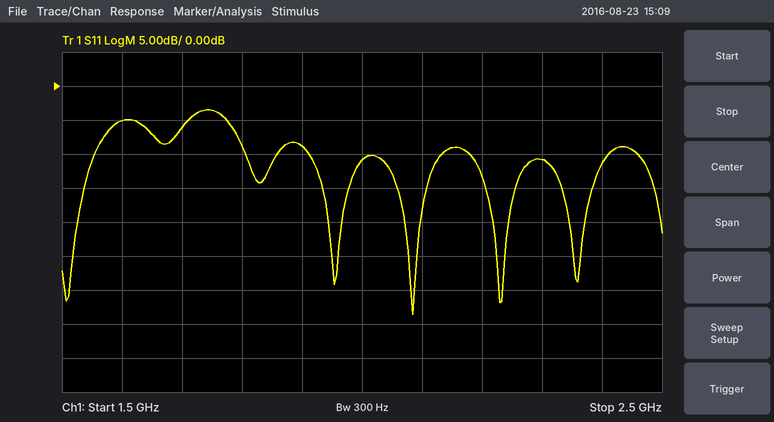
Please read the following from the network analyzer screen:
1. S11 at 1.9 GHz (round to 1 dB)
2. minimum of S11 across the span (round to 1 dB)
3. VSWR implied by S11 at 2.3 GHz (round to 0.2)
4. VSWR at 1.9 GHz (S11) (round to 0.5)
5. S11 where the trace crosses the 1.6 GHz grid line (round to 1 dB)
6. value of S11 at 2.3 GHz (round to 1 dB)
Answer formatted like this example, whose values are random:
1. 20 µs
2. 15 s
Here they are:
1. -9 dB
2. -34 dB
3. 1.8
4. 2.0
5. -5 dB
6. -11 dB
